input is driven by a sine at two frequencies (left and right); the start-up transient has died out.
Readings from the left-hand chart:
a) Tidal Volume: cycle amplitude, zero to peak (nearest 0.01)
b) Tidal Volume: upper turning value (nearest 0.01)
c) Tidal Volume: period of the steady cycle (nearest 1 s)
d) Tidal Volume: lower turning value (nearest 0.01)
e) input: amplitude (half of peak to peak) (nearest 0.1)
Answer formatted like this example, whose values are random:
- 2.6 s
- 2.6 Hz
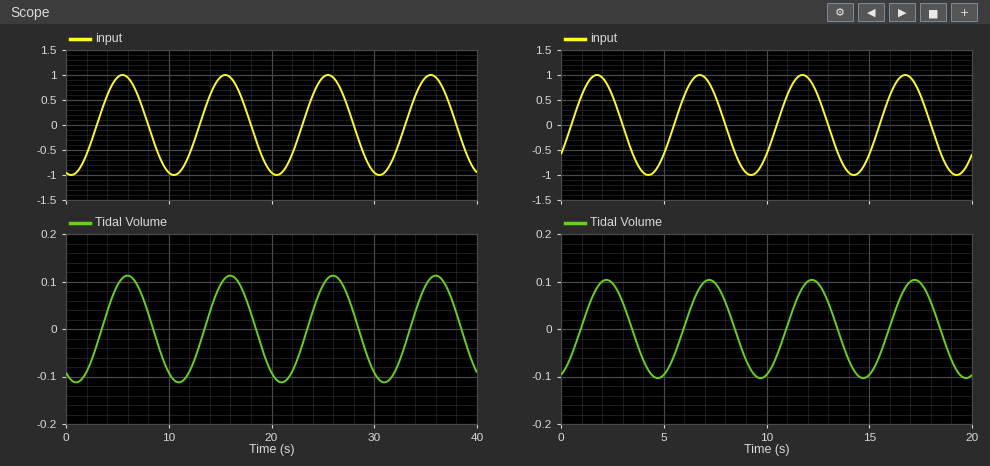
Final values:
- 0.11
- 0.11
- 10 s
- -0.11
- 1.0
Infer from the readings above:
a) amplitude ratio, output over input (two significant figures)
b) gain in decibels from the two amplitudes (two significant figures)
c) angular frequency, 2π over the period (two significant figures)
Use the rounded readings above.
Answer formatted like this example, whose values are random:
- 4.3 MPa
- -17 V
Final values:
- 0.11
- -19 dB
- 0.63 rad/s
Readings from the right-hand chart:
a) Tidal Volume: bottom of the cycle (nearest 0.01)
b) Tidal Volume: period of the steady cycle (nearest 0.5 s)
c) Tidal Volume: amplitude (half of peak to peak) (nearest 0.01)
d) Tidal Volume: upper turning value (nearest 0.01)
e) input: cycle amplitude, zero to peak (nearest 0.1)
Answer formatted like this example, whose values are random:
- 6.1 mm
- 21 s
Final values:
- -0.10
- 5.0 s
- 0.10
- 0.10
- 1.0
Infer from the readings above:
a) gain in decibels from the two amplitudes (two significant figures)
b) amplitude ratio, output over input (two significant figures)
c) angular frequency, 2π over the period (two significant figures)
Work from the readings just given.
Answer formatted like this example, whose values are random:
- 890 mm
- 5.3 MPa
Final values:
- -20 dB
- 0.10
- 1.3 rad/s
